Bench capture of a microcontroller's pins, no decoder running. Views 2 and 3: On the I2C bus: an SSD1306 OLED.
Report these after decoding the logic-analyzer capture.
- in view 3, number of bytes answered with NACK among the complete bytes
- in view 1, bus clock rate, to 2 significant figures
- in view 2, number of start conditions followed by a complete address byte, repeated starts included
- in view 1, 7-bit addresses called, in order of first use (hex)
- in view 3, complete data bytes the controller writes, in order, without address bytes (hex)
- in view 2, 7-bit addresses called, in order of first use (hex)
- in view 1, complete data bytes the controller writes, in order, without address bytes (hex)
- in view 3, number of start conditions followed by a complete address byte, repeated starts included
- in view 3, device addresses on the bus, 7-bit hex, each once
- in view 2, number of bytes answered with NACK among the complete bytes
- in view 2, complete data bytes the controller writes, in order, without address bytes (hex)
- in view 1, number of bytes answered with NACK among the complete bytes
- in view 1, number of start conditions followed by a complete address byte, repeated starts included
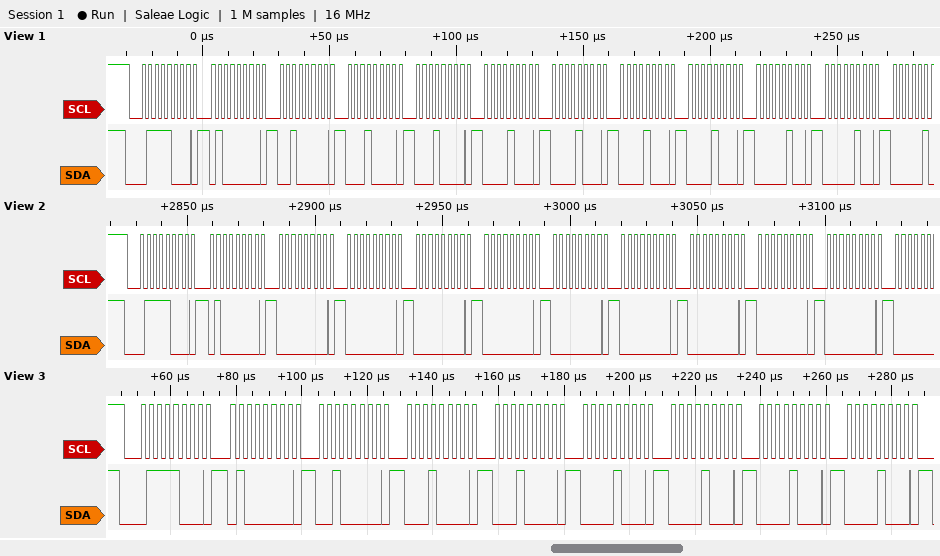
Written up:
0
400 kHz
1
0x3C
40 20 10 10 08 08 08 08
0x3C
40 20 10 10 08 08 08 08 04 04
1
0x3C
0
40 00 00 00 00 00 00 00 00 00
0
1
